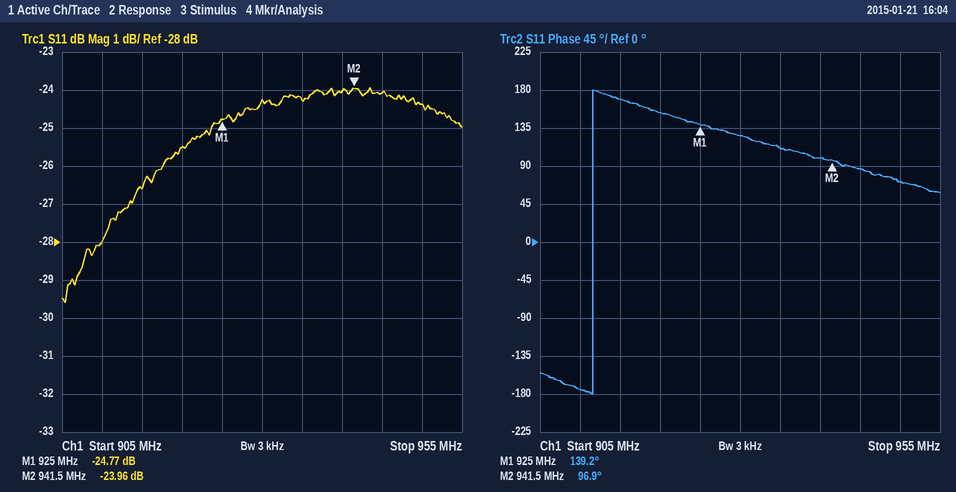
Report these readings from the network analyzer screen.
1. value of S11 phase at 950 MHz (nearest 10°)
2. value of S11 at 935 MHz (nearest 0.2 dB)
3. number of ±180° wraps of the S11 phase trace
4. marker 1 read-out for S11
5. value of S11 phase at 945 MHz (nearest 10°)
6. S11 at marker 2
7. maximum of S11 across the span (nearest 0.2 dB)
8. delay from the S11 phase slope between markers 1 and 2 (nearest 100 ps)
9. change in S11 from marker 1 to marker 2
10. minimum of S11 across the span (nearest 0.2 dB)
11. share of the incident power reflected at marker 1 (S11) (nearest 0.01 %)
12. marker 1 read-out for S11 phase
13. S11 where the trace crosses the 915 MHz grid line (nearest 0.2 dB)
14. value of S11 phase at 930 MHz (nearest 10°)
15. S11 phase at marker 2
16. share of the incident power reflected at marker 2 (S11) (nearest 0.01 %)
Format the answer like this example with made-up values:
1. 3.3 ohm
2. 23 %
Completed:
1. 70°
2. -24.2 dB
3. 1
4. -24.77 dB
5. 90°
6. -23.96 dB
7. -24.0 dB
8. 7.1 ns
9. 0.81 dB
10. -29.6 dB
11. 0.33 %
12. 139.2°
13. -26.6 dB
14. 130°
15. 96.9°
16. 0.40 %
